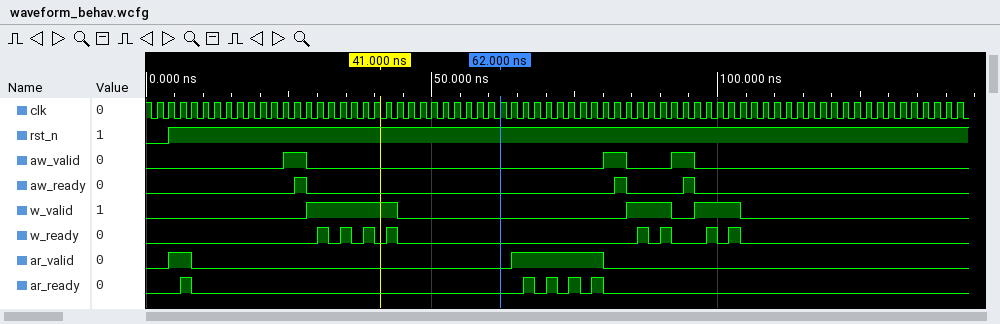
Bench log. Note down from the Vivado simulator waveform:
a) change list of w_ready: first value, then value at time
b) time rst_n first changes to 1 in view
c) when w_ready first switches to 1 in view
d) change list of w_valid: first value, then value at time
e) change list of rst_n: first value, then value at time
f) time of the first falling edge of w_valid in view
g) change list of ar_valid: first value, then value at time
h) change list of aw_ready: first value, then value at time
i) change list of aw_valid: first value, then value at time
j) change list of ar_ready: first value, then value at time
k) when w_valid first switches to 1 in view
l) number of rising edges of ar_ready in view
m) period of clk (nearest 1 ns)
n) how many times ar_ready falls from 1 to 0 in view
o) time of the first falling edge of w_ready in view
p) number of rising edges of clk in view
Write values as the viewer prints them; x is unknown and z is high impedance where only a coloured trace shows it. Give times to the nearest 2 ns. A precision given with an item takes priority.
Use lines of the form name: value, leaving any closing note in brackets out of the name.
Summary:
change list of w_ready: first value, then value at time: 0, 1 at 30 ns, 0 at 32 ns, 1 at 34 ns, 0 at 36 ns, 1 at 38 ns, 0 at 40 ns, 1 at 42 ns, 0 at 44 ns, 1 at 86 ns, 0 at 88 ns, 1 at 90 ns, 0 at 92 ns, 1 at 98 ns, 0 at 100 ns, 1 at 102 ns, 0 at 104 ns
time rst_n first changes to 1 in view: 4 ns
when w_ready first switches to 1 in view: 30 ns
change list of w_valid: first value, then value at time: 0, 1 at 28 ns, 0 at 44 ns, 1 at 84 ns, 0 at 92 ns, 1 at 96 ns, 0 at 104 ns
change list of rst_n: first value, then value at time: 0, 1 at 4 ns
time of the first falling edge of w_valid in view: 44 ns
change list of ar_valid: first value, then value at time: 0, 1 at 4 ns, 0 at 8 ns, 1 at 64 ns, 0 at 80 ns
change list of aw_ready: first value, then value at time: 0, 1 at 26 ns, 0 at 28 ns, 1 at 82 ns, 0 at 84 ns, 1 at 94 ns, 0 at 96 ns
change list of aw_valid: first value, then value at time: 0, 1 at 24 ns, 0 at 28 ns, 1 at 80 ns, 0 at 84 ns, 1 at 92 ns, 0 at 96 ns
change list of ar_ready: first value, then value at time: 0, 1 at 6 ns, 0 at 8 ns, 1 at 66 ns, 0 at 68 ns, 1 at 70 ns, 0 at 72 ns, 1 at 74 ns, 0 at 76 ns, 1 at 78 ns, 0 at 80 ns
when w_valid first switches to 1 in view: 28 ns
number of rising edges of ar_ready in view: 5
period of clk: 2 ns
how many times ar_ready falls from 1 to 0 in view: 5
time of the first falling edge of w_ready in view: 32 ns
number of rising edges of clk in view: 71
